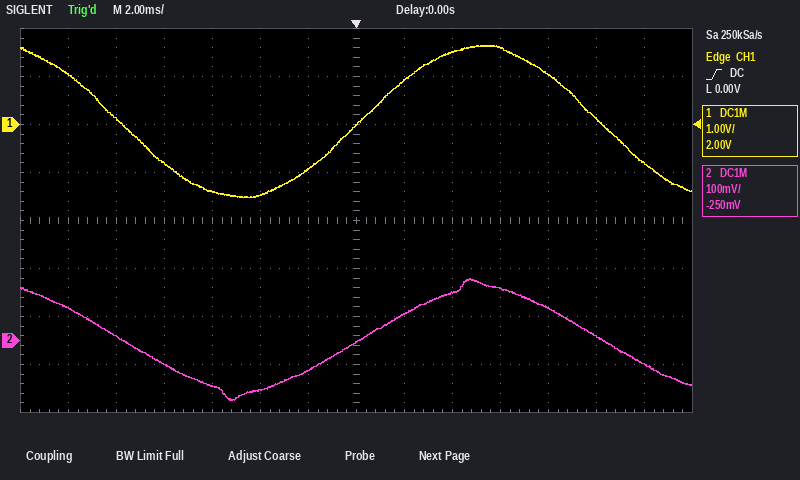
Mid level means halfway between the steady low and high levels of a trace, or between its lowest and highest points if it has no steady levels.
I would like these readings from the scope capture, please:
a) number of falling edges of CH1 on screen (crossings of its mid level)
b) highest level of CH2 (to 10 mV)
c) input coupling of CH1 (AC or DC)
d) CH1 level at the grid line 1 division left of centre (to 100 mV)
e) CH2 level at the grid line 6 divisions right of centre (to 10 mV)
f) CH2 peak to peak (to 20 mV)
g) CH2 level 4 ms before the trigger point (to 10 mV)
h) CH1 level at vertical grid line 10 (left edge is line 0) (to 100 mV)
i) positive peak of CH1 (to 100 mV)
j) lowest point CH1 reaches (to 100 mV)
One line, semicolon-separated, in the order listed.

2; 130 mV; DC; -900 mV; -50 mV; 260 mV; -100 mV; 1.6 V; 1.6 V; -1.5 V
